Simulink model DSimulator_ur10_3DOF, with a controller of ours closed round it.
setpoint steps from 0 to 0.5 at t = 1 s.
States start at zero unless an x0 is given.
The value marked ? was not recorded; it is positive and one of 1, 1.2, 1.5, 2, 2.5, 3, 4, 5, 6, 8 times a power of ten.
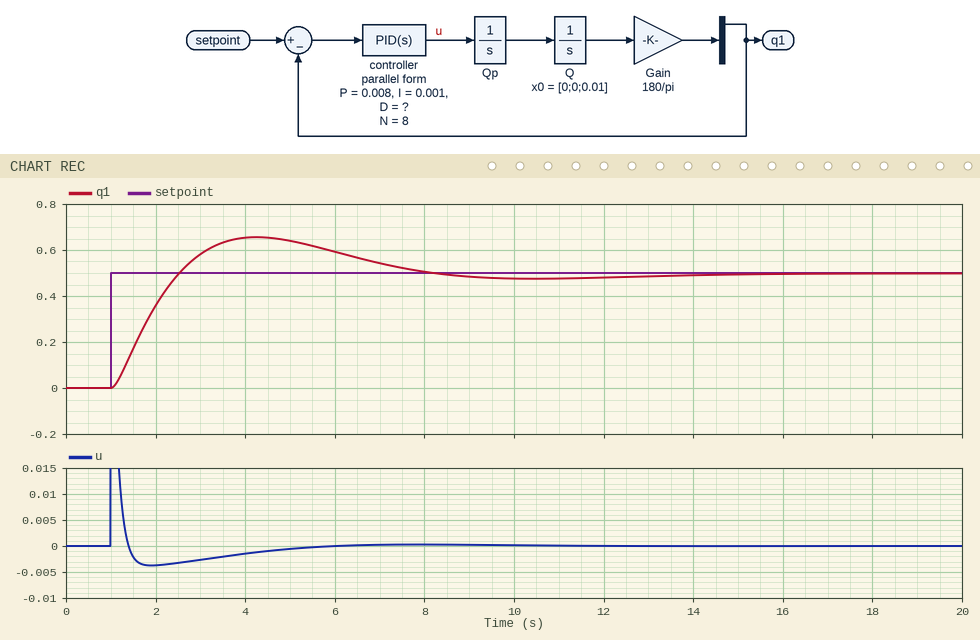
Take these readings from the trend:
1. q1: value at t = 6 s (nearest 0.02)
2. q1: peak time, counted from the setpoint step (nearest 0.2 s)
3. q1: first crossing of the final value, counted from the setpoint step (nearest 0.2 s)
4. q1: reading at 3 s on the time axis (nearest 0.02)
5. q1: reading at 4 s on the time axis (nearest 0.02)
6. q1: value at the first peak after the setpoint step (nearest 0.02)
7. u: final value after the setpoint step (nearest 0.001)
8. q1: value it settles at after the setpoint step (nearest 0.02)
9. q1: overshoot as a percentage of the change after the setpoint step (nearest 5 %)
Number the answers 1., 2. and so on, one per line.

1. 0.60
2. 3.2 s
3. 1.6 s
4. 0.58
5. 0.66
6. 0.66
7. 0.000
8. 0.50
9. 30 %
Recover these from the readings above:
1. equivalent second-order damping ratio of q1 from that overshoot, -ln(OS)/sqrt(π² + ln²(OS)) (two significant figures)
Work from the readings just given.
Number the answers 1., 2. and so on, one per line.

1. 0.36
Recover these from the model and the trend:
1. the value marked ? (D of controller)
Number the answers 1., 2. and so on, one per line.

1. 0.015
